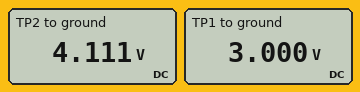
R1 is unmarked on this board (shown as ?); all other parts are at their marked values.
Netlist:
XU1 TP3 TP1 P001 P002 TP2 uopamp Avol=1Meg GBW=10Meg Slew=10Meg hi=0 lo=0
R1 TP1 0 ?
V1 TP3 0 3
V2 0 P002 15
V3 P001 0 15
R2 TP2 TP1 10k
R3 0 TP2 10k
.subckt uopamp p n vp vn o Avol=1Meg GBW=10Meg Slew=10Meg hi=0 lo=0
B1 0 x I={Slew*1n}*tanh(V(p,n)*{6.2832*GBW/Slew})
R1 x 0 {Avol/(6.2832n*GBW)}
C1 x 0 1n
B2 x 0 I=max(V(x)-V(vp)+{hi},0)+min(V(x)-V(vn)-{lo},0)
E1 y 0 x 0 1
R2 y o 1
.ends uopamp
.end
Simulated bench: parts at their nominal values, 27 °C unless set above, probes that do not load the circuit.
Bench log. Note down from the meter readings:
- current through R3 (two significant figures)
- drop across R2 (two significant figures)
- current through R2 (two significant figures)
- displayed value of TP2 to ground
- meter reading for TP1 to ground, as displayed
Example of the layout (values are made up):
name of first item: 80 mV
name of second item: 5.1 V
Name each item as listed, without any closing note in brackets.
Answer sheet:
current through R3: 410 µA
drop across R2: 1.1 V
current through R2: 110 µA
displayed value of TP2 to ground: 4.111 V
meter reading for TP1 to ground, as displayed: 3.000 V
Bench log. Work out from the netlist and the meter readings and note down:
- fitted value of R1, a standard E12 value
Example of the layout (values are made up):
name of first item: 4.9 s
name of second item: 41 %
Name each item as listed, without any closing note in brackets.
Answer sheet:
fitted value of R1, a standard E12 value: 27 kΩ
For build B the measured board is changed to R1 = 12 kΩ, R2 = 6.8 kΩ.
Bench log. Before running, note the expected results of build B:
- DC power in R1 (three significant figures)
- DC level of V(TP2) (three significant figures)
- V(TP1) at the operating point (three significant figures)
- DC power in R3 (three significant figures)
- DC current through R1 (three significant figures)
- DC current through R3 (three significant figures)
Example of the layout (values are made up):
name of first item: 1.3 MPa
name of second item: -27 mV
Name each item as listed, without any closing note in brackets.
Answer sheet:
DC power in R1: 750 µW
DC level of V(TP2): 4.70 V
V(TP1) at the operating point: 3.00 V
DC power in R3: 2.21 mW
DC current through R1: 250 µA
DC current through R3: 470 µA
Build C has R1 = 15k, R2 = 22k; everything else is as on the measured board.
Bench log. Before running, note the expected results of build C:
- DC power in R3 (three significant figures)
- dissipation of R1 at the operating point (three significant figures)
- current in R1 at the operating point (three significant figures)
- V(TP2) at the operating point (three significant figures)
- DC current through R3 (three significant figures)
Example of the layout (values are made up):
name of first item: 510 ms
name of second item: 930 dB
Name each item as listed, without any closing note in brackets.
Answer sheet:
DC power in R3: 5.48 mW
dissipation of R1 at the operating point: 600 µW
current in R1 at the operating point: 200 µA
V(TP2) at the operating point: 7.40 V
DC current through R3: 740 µA
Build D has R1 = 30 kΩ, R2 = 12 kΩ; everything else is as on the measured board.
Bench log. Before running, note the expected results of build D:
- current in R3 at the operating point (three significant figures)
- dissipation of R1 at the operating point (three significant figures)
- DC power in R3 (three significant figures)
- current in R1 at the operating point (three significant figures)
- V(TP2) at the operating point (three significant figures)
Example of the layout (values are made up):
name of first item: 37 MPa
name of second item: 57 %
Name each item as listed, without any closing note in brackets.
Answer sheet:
current in R3 at the operating point: 420 µA
dissipation of R1 at the operating point: 300 µW
DC power in R3: 1.76 mW
current in R1 at the operating point: 100 µA
V(TP2) at the operating point: 4.20 V
